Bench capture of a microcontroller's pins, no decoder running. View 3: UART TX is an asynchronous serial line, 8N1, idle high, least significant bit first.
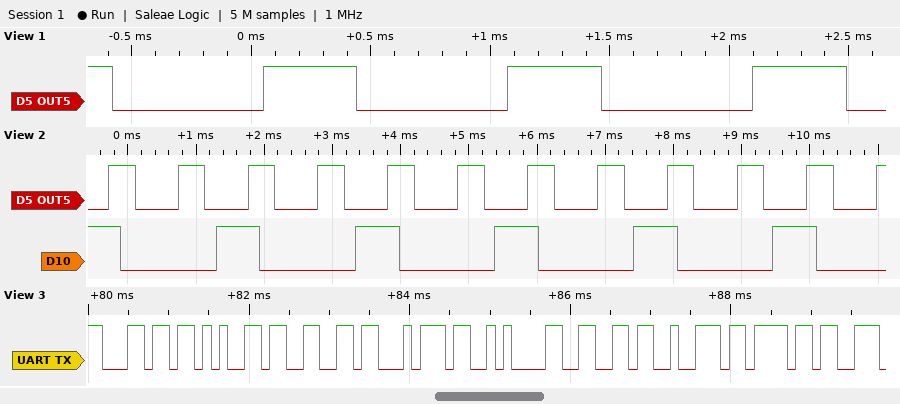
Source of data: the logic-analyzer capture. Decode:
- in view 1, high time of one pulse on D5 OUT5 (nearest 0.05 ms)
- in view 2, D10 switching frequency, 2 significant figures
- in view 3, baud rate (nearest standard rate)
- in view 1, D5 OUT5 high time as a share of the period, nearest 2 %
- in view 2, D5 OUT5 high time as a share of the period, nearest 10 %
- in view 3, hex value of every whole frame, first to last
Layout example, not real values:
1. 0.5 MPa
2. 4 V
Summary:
1. 0.40 ms
2. 490 Hz
3. 9600 baud
4. 38 %
5. 40 %
6. 6C 65 66 74 0A 66 72 6F
